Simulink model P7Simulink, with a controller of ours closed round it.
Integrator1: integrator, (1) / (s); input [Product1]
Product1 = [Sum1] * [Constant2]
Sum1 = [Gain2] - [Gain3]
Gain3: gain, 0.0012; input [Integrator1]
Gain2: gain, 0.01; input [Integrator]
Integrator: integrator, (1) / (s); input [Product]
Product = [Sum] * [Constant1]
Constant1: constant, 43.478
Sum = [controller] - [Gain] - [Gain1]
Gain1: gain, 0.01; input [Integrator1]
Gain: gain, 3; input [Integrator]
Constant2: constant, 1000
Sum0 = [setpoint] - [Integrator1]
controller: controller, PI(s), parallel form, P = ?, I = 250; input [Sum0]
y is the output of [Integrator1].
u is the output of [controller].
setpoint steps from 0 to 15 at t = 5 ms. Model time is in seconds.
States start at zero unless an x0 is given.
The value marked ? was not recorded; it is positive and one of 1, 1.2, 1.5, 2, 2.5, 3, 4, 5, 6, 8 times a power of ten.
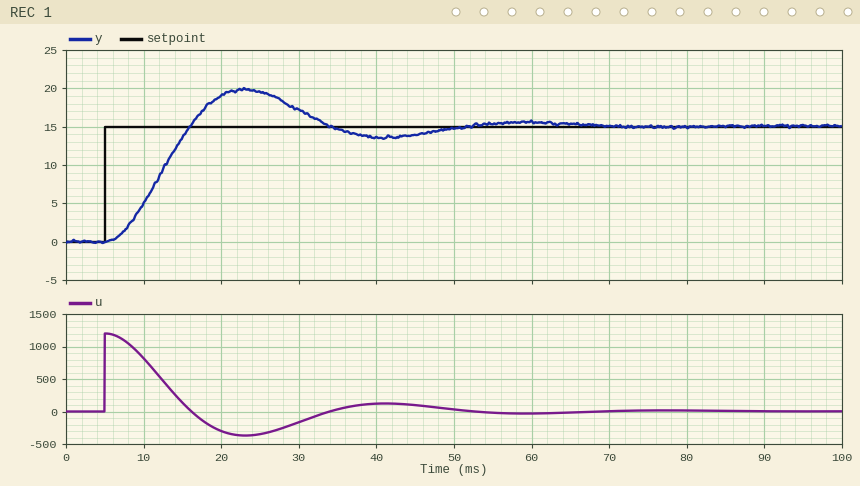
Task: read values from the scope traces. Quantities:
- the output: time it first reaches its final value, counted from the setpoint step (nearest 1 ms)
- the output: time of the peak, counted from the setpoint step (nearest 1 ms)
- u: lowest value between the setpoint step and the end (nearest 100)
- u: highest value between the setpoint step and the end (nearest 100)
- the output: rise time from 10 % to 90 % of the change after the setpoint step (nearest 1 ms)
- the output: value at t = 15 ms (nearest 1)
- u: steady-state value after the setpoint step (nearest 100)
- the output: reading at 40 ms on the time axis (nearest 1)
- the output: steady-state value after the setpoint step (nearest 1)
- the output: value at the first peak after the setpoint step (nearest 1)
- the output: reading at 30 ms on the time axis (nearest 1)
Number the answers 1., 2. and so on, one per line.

1. 11 ms
2. 18 ms
3. -400
4. 1200
5. 7 ms
6. 14
7. 0
8. 14
9. 15
10. 20
11. 17
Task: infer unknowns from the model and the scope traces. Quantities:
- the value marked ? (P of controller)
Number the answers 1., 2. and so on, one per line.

1. 80
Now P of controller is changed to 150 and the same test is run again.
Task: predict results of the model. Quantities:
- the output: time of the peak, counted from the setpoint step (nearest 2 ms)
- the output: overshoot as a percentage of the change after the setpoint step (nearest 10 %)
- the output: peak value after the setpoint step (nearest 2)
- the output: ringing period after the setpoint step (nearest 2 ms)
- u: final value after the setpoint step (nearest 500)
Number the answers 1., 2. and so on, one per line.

1. 12 ms
2. 40 %
3. 22
4. 26 ms
5. 0
